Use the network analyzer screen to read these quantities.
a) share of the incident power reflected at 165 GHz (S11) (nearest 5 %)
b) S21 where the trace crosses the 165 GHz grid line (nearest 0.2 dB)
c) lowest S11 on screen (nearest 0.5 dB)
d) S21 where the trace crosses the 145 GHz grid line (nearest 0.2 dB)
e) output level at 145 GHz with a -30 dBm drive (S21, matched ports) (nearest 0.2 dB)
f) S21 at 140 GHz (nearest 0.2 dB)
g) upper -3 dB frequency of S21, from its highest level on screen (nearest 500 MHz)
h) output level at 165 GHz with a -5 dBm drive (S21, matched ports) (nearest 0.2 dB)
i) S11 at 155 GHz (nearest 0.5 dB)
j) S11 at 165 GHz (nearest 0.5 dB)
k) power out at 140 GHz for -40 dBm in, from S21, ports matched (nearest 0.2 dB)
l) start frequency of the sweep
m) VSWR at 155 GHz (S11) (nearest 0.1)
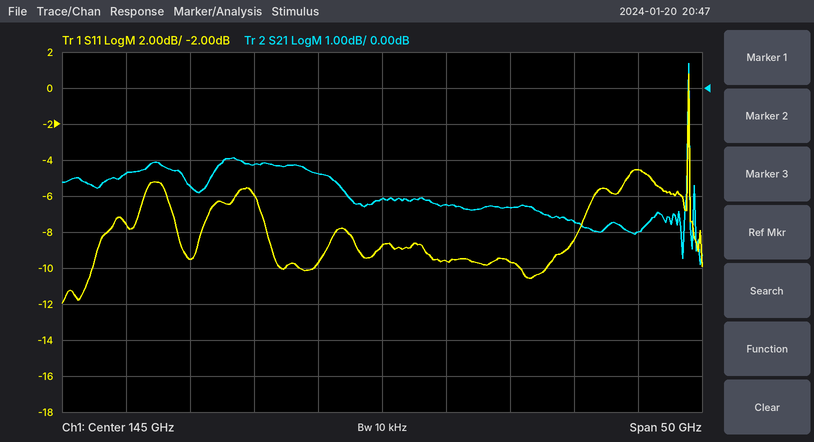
35 %
-4.0 dB
-12.0 dB
-3.0 dB
-33.0 dBm
-2.4 dB
169.0 GHz
-9.0 dBm
-9.5 dB
-4.5 dB
-42.4 dBm
120 GHz
2.0
